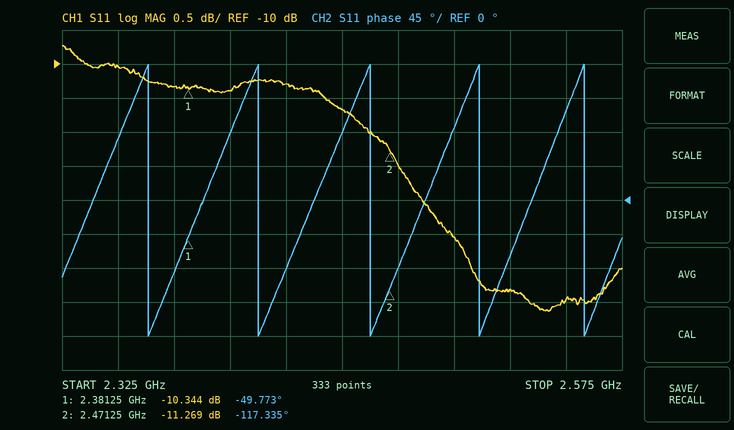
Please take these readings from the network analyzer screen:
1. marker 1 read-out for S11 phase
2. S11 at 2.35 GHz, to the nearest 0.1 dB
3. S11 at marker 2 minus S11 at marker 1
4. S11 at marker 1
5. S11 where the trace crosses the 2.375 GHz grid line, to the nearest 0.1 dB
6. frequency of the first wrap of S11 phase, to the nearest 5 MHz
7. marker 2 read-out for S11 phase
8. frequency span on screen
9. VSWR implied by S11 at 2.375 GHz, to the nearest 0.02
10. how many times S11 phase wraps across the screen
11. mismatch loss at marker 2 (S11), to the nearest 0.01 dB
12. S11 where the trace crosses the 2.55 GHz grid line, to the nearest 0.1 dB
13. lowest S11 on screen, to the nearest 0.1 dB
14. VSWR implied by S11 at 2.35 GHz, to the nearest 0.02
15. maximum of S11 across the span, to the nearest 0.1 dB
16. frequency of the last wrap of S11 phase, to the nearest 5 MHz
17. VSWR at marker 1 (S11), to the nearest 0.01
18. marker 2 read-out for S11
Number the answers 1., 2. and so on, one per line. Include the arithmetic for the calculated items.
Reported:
1. -49.773°
2. -10.0 dB
3. -11.269 − (-10.344) = -0.925 dB
4. -10.344 dB
5. -10.3 dB
6. 2.365 GHz
7. -117.335°
8. 250 MHz
9. |Γ| = 10^(-10.3/20) = 0.3055; VSWR = (1 + 0.3055)/(1 − 0.3055) ≈ 1.88
10. 5
11. −10 log10(1 − 10^(-11.269/10)) ≈ 0.34 dB
12. -13.5 dB
13. -13.6 dB
14. |Γ| = 10^(-10/20) = 0.3162; VSWR = (1 + 0.3162)/(1 − 0.3162) ≈ 1.92
15. -9.7 dB
16. 2.560 GHz
17. (1 + 0.3039)/(1 − 0.3039) ≈ 1.87
18. -11.269 dB
